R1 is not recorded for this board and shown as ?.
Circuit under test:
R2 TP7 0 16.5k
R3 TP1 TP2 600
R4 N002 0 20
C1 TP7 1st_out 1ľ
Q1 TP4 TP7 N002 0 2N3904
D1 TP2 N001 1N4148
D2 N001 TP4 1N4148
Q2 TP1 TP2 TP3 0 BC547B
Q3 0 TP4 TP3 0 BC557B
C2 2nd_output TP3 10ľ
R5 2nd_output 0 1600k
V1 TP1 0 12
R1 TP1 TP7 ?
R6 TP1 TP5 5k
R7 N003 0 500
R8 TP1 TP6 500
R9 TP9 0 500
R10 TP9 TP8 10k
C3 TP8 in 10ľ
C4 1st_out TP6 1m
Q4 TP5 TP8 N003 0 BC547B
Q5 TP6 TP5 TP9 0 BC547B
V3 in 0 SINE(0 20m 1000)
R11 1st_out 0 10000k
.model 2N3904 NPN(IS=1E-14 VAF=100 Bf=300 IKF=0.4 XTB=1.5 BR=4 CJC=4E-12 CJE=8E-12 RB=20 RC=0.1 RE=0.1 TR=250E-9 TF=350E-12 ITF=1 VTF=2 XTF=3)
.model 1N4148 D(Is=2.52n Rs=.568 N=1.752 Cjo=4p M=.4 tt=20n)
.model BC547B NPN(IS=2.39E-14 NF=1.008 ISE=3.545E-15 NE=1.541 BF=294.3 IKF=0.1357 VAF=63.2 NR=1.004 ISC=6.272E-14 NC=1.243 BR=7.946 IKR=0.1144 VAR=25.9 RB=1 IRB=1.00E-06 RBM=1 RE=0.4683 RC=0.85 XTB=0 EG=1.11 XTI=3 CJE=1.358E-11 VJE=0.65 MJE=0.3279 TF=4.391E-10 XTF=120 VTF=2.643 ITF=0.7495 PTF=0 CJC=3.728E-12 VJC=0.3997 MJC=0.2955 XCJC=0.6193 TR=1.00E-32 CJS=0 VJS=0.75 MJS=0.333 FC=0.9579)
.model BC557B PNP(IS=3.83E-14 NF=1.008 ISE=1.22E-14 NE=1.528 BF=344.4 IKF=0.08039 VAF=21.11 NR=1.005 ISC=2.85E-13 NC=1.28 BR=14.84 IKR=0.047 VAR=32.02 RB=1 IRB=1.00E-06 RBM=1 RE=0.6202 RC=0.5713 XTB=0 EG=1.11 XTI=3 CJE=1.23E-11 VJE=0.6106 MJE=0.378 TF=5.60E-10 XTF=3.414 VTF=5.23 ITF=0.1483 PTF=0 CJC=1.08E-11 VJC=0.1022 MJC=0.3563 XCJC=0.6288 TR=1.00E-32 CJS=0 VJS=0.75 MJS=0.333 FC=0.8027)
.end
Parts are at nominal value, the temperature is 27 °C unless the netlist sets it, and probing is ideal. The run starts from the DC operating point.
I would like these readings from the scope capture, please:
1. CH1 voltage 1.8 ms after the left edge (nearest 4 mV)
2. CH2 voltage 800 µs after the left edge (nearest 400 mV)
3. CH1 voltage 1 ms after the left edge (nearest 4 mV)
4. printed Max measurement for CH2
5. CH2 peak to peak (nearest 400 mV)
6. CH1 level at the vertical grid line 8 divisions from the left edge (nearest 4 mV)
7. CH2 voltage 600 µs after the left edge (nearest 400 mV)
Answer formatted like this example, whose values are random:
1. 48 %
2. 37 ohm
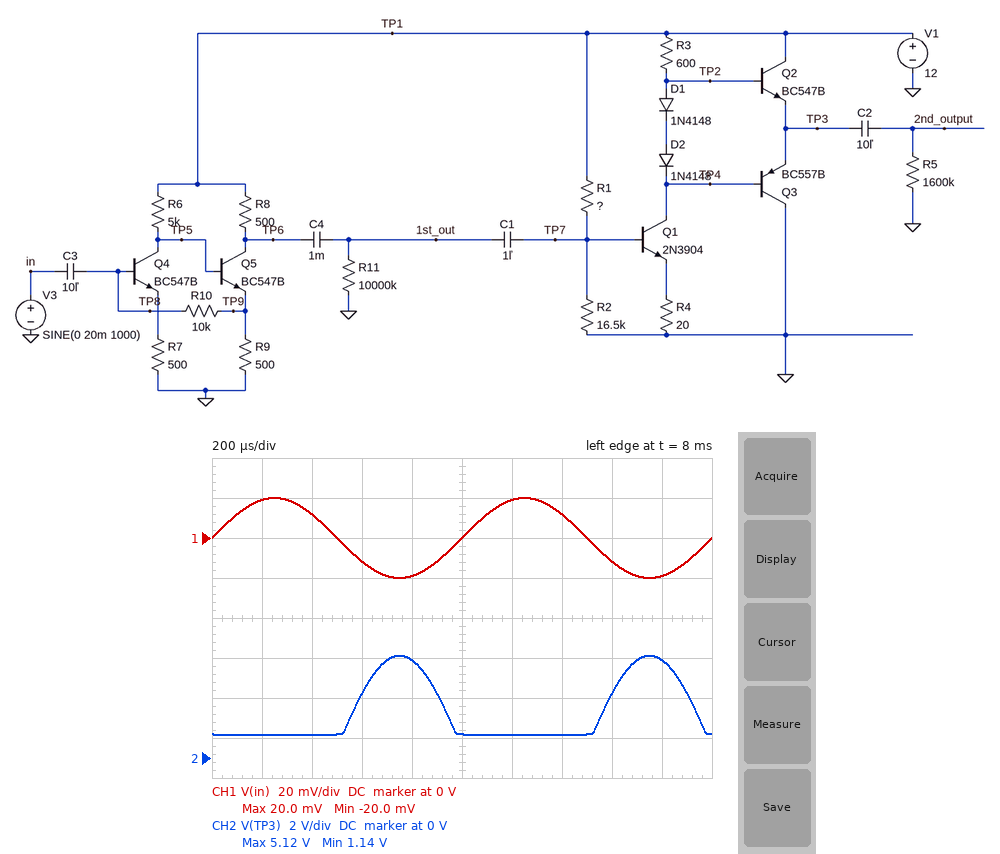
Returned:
1. -20 mV
2. 4.8 V
3. 0 V
4. 5.12 V
5. 4.0 V
6. -12 mV
7. 3.2 V
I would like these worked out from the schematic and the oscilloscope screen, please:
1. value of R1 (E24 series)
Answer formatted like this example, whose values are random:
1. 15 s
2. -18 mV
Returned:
1. 62 kΩ
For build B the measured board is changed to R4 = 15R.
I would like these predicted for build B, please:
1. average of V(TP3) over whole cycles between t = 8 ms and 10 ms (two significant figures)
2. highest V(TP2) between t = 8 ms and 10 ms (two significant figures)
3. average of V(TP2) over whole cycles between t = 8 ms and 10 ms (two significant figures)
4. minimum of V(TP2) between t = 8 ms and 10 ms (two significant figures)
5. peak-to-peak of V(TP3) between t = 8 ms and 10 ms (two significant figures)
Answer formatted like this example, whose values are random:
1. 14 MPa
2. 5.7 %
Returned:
1. 2.5 V
2. 6.6 V
3. 3.2 V
4. 1.8 V
5. 4.9 V
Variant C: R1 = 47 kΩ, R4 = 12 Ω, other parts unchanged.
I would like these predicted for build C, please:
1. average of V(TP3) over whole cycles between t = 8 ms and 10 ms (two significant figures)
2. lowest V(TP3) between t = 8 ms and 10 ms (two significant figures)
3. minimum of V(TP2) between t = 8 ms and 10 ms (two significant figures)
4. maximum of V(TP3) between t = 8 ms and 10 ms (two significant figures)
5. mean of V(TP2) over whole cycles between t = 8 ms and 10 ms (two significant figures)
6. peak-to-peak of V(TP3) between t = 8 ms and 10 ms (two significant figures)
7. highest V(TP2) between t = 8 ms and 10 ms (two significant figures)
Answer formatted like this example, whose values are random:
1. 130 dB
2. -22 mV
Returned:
1. 2.2 V
2. 1.0 V
3. 1.7 V
4. 5.6 V
5. 2.9 V
6. 4.6 V
7. 6.3 V
